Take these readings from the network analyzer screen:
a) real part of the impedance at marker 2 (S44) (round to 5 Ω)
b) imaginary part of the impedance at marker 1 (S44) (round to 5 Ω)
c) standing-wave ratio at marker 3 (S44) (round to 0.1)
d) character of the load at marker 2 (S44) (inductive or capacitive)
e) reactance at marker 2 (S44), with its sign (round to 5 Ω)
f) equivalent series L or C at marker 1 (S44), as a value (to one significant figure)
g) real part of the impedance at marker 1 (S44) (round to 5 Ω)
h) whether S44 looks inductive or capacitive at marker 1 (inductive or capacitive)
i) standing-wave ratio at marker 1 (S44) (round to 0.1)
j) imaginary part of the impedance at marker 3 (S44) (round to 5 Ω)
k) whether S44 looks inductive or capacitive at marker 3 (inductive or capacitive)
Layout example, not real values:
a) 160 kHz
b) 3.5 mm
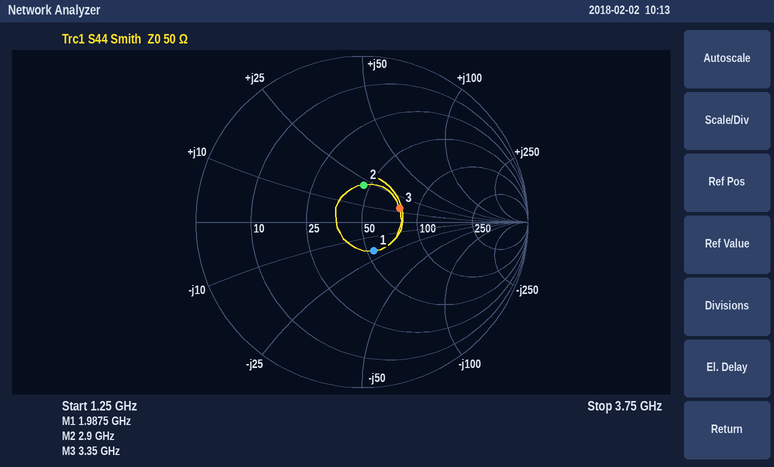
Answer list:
a) 45 Ω
b) -20 Ω
c) 1.6
d) inductive
e) +20 Ω
f) 4 pF
g) 55 Ω
h) capacitive
i) 1.5
j) +15 Ω
k) inductive
